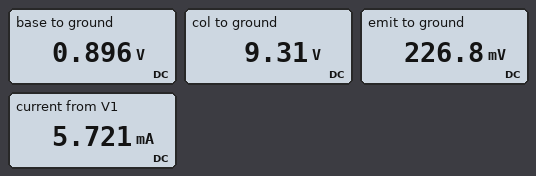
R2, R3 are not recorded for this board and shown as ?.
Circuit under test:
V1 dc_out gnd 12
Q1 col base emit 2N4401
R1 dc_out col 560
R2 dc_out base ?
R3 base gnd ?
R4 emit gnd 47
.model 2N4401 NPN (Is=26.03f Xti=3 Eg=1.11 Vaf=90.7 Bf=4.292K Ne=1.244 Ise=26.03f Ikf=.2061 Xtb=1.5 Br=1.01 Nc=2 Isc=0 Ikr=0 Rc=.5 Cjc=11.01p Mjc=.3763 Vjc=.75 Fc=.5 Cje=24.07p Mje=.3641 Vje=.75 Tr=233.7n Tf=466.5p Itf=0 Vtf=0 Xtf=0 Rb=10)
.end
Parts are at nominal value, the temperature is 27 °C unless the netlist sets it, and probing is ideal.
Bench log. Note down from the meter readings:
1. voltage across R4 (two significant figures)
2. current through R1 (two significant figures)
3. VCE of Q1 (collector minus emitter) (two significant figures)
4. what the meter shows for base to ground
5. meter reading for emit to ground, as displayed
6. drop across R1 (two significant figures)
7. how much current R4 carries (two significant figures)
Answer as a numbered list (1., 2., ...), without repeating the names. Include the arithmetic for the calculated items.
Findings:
1. 226.8 mV = 230 mV
2. (12 V - 9.31 V) / 560 Ω = 4.8 mA
3. 9.31 V - 226.8 mV = 9.1 V
4. 0.896 V
5. 226.8 mV
6. 12 V - 9.31 V = 2.7 V
7. (226.8 mV) / 47 Ω = 4.8 mA
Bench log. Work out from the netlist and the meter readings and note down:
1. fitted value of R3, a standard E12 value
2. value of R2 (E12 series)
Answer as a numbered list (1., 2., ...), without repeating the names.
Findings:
1. 1 kΩ
2. 12 kΩ
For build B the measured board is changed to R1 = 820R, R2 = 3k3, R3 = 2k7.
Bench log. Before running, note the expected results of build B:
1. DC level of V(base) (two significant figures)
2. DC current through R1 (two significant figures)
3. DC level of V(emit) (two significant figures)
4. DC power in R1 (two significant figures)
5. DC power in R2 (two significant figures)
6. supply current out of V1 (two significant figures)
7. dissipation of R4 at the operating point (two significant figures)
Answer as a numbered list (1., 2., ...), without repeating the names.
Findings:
1. 1.5 V
2. 14 mA
3. 760 mV
4. 150 mW
5. 33 mW
6. 17 mA
7. 12 mW
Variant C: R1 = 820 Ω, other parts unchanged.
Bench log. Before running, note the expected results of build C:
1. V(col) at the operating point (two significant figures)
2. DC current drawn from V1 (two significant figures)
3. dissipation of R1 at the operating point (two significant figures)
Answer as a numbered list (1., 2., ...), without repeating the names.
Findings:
1. 8.1 V
2. 5.7 mA
3. 19 mW
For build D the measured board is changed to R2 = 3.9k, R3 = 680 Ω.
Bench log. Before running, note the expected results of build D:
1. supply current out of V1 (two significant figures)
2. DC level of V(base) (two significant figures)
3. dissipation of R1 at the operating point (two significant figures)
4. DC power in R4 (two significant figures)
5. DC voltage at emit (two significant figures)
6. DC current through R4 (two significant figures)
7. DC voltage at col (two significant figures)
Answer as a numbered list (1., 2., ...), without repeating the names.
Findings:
1. 22 mA
2. 1.6 V
3. 210 mW
4. 18 mW
5. 930 mV
6. 20 mA
7. 1.1 V
